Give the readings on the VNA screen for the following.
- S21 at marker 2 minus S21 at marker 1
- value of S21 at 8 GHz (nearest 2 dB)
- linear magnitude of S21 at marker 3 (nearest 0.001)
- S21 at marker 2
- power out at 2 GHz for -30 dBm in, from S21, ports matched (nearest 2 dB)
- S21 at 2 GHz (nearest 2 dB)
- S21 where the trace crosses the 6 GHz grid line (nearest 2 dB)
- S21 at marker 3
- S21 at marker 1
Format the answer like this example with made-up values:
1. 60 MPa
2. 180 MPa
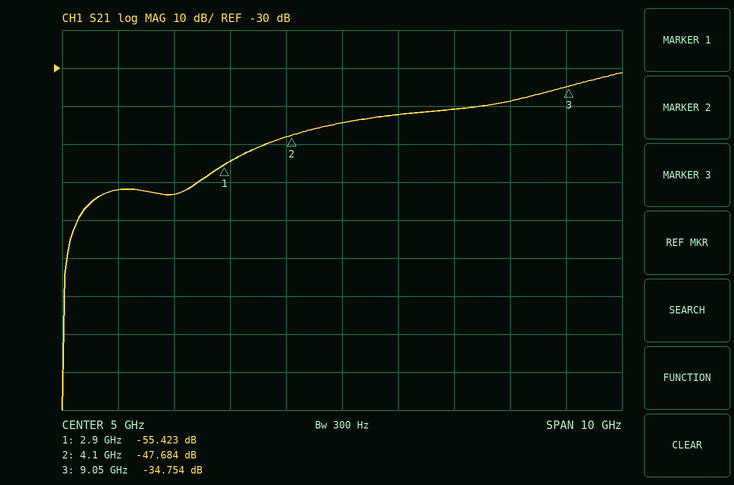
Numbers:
1. 7.739 dB
2. -38 dB
3. 0.018
4. -47.684 dB
5. -94 dBm
6. -64 dB
7. -42 dB
8. -34.754 dB
9. -55.423 dB
